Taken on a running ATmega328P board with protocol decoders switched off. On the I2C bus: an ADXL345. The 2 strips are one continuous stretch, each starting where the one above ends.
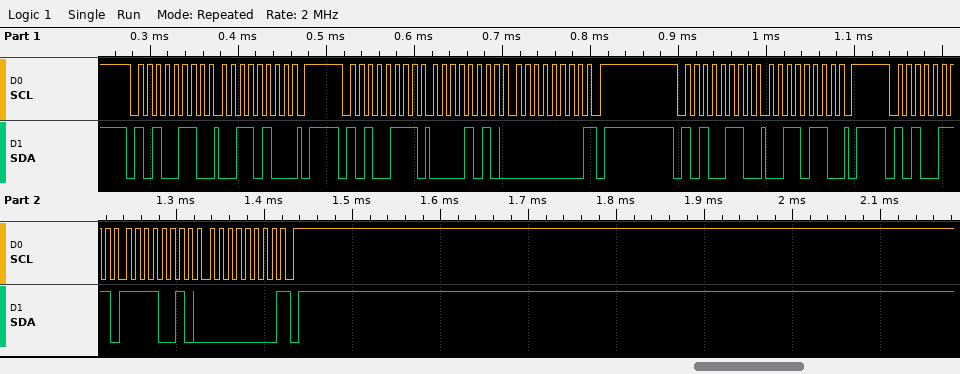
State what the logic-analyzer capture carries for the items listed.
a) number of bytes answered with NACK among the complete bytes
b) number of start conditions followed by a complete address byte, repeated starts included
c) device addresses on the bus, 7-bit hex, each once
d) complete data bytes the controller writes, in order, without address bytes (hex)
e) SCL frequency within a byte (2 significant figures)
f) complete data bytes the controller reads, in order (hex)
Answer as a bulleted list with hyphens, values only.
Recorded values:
- 2
- 4
- 0x53
- 34 36
- 100 kHz
- 0A 00 F2 00
